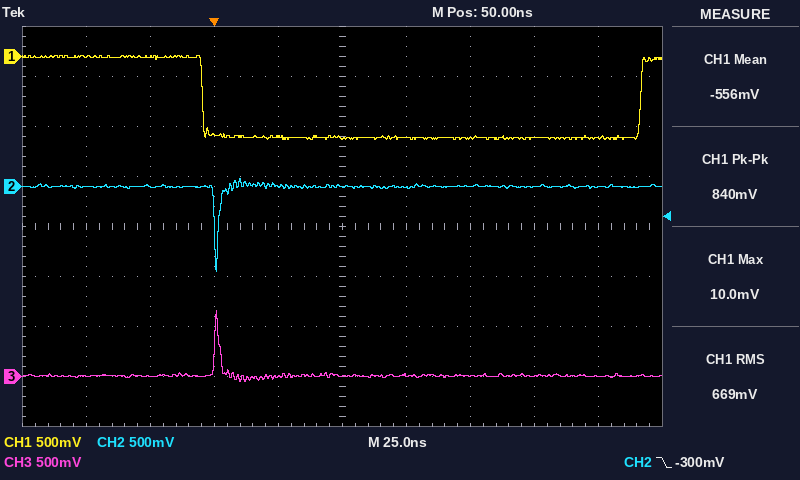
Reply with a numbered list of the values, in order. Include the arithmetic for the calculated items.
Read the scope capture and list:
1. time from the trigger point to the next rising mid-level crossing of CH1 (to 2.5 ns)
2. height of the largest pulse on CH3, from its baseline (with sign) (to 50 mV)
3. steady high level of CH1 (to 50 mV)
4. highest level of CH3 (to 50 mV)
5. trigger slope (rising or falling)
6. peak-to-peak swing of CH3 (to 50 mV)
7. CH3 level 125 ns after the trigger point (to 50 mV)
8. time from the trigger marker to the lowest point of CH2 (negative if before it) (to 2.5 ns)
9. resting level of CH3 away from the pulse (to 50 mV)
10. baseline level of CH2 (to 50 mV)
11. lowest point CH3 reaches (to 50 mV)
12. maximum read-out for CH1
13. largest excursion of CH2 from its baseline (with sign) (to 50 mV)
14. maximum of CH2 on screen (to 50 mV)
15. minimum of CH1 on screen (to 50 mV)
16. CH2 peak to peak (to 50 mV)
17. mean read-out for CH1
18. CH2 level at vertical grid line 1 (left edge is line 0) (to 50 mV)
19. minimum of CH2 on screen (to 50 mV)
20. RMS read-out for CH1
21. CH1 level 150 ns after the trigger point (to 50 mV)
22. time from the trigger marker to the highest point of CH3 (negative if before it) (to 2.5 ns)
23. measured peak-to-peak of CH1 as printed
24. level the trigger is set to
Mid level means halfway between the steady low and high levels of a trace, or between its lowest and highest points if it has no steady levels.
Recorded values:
1. 167.5 ns
2. 650 mV − (0 mV) = +650 mV
3. 0 mV
4. 650 mV
5. falling
6. 650 mV − (-50 mV) = 700 mV
7. 0 mV
8. 0.0 ns
9. 0 mV
10. 0 mV
11. -50 mV
12. 10.0 mV
13. -850 mV − (0 mV) = -850 mV
14. 100 mV
15. -850 mV
16. 100 mV − (-850 mV) = 950 mV
17. -556 mV
18. 0 mV
19. -850 mV
20. 669 mV
21. -800 mV
22. 0.0 ns
23. 840 mV
24. -300 mV
